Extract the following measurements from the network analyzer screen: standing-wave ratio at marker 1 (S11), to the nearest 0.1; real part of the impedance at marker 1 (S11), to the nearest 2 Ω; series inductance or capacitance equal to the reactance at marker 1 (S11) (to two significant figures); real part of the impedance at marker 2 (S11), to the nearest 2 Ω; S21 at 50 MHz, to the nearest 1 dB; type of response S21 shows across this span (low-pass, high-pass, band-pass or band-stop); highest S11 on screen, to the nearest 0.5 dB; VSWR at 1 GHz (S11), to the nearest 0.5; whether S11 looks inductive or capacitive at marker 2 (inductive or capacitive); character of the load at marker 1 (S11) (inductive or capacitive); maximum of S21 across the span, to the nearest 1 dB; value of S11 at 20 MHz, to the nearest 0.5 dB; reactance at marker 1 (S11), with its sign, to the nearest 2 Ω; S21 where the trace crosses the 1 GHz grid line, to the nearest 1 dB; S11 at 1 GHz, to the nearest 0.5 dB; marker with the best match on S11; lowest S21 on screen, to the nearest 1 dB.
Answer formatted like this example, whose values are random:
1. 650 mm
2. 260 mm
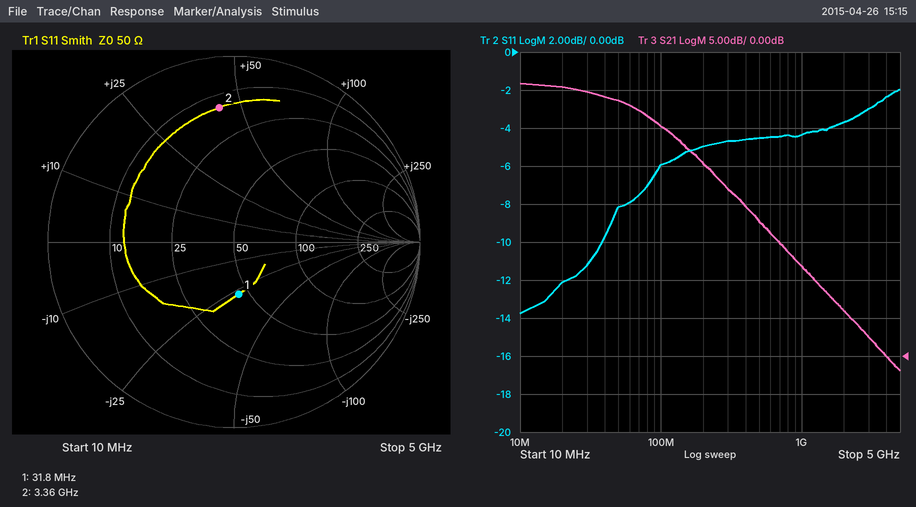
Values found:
1. 1.8
2. 44 Ω
3. 180 pF
4. 14 Ω
5. 34 dB
6. low-pass
7. -2.0 dB
8. 4.0
9. inductive
10. capacitive
11. 36 dB
12. -12.0 dB
13. -28 Ω
14. 12 dB
15. -4.5 dB
16. marker 1
17. -2 dB
